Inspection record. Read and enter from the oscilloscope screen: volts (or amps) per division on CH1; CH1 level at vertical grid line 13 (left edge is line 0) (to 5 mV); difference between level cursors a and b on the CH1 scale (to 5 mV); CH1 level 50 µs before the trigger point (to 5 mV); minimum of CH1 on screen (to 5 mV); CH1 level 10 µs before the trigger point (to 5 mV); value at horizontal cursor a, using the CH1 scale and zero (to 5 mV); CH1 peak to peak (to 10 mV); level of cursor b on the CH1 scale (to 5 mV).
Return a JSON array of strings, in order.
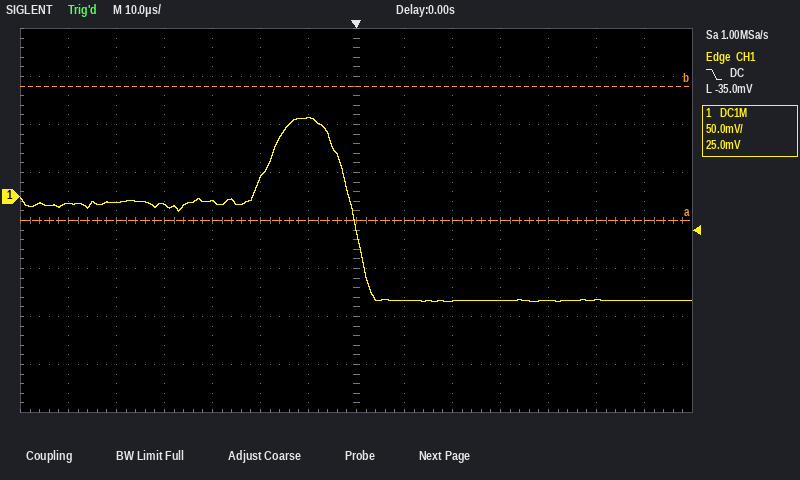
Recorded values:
["50 mV", "-110 mV", "140 mV", "-5 mV", "-110 mV", "80 mV", "-25 mV", "190 mV", "115 mV"]
